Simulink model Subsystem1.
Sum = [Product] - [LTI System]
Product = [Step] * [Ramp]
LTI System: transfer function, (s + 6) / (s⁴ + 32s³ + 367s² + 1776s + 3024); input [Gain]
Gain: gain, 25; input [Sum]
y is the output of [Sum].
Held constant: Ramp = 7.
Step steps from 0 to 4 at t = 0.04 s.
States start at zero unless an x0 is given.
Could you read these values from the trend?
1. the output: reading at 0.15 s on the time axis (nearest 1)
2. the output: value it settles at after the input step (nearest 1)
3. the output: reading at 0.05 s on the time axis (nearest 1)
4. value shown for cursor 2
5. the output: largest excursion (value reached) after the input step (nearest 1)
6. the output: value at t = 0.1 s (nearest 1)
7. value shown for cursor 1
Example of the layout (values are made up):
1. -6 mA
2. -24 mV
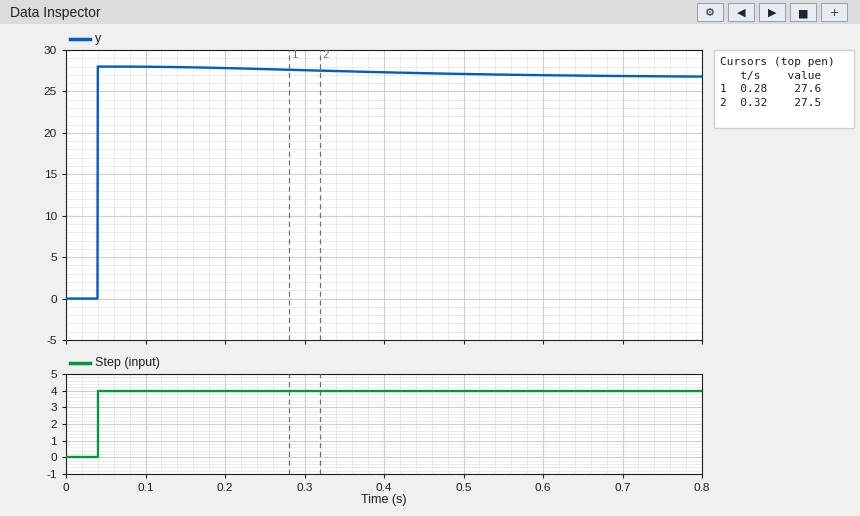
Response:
1. 28
2. 27
3. 28
4. 27.5
5. 28
6. 28
7. 27.6
